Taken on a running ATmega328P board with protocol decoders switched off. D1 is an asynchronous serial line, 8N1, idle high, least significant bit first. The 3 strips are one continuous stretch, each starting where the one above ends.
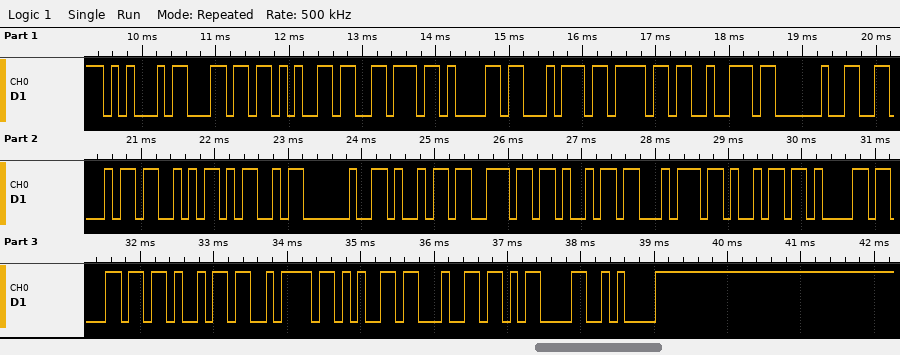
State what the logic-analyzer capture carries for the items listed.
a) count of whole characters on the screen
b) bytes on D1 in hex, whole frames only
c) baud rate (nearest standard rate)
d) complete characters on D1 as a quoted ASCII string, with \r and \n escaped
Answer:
26
45 6C 65 76 61 74 6F 72 20 46 53 4D 20 69 6E 69 74 69 61 6C 69 7A 65 64 0D 0A
9600 baud
"Elevator FSM initialized\r\n"
